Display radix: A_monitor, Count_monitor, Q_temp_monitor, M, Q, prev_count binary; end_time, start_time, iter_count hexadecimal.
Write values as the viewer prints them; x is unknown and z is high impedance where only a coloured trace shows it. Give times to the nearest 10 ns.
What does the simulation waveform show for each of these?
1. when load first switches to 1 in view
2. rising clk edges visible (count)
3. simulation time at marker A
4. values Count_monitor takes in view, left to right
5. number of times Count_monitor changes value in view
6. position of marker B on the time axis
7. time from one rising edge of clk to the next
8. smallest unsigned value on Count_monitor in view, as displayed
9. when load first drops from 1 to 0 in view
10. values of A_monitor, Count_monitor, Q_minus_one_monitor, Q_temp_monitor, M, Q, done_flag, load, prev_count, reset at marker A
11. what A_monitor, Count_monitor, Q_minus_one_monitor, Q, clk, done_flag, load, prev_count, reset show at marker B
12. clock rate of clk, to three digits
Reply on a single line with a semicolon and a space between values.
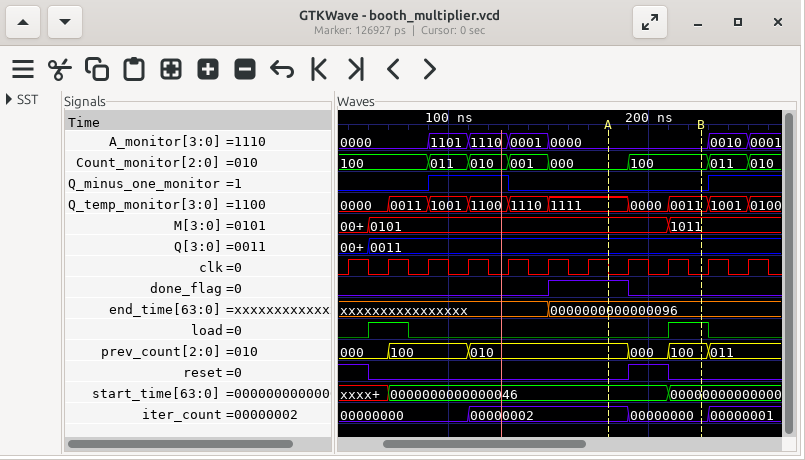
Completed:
60 ns; 11; 180 ns; 100, 011, 010, 001, 000, 100, 011, 010; 7; 230 ns; 20 ns; 000; 80 ns; A_monitor=0000, Count_monitor=000, Q_minus_one_monitor=0, Q_temp_monitor=1111, M=0101, Q=0011, done_flag=1, load=0, prev_count=010, reset=0; A_monitor=0000, Count_monitor=100, Q_minus_one_monitor=0, Q=0011, clk=0, done_flag=0, load=1, prev_count=100, reset=0; 50.0 MHz
